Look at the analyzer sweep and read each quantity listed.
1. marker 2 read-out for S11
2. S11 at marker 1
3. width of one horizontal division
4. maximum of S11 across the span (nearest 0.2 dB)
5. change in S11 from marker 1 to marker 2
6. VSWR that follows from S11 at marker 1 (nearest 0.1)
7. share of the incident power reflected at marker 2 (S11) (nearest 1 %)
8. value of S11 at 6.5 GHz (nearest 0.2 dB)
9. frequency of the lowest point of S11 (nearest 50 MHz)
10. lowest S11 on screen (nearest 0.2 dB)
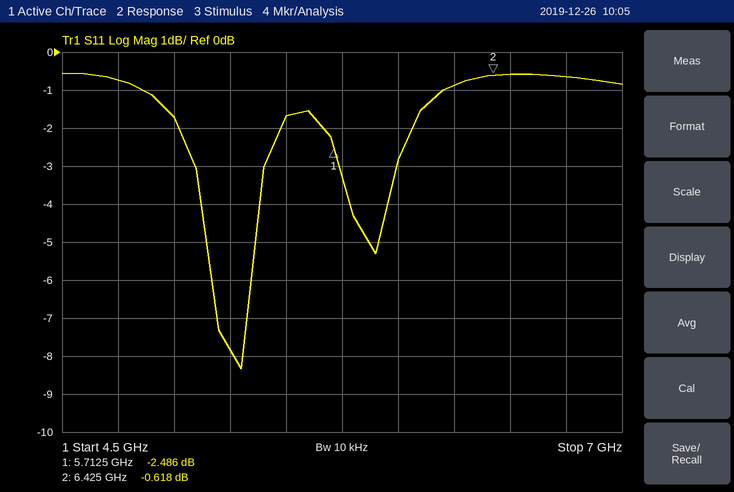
-0.618 dB
-2.486 dB
250 MHz
-0.6 dB
1.868 dB
7.0
87 %
-0.6 dB
5.30 GHz
-8.4 dB
